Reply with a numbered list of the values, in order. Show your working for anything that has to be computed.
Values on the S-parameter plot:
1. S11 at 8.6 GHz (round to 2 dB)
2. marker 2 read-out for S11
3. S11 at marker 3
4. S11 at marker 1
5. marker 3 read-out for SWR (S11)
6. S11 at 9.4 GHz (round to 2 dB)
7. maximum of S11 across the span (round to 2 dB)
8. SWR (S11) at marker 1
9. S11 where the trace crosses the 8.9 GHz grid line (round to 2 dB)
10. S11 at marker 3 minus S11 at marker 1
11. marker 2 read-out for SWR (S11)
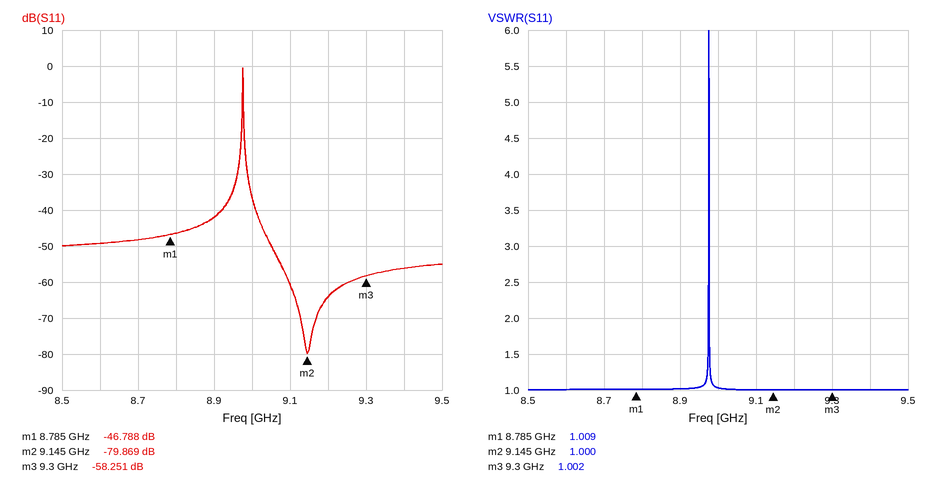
1. -50 dB
2. -79.869 dB
3. -58.251 dB
4. -46.788 dB
5. 1.002
6. -56 dB
7. 0 dB
8. 1.009
9. -42 dB
10. -58.251 − (-46.788) = -11.463 dB
11. 1.000
